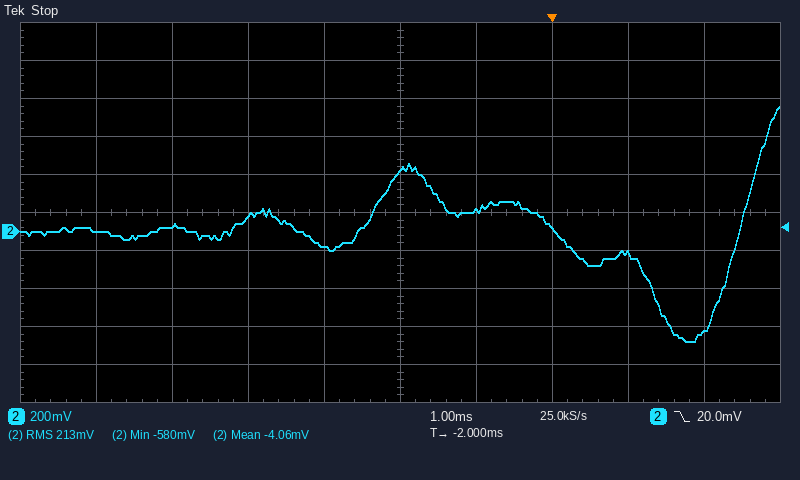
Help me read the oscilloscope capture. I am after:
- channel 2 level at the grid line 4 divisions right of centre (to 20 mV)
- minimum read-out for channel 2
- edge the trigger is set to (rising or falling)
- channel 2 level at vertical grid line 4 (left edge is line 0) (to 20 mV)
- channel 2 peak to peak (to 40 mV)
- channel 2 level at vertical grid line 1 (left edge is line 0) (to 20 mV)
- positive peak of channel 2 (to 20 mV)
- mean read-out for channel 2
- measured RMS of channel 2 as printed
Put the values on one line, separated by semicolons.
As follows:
-520 mV; -580 mV; falling; -80 mV; 1.24 V; 0 mV; 660 mV; -4.06 mV; 213 mV
